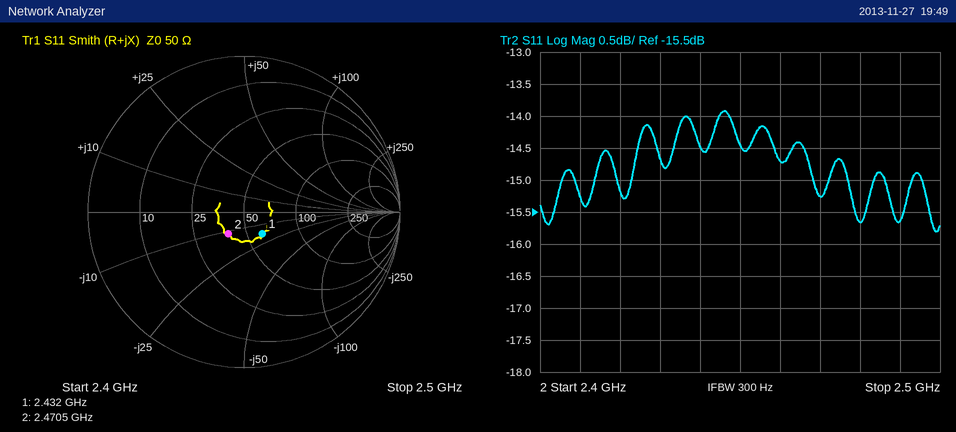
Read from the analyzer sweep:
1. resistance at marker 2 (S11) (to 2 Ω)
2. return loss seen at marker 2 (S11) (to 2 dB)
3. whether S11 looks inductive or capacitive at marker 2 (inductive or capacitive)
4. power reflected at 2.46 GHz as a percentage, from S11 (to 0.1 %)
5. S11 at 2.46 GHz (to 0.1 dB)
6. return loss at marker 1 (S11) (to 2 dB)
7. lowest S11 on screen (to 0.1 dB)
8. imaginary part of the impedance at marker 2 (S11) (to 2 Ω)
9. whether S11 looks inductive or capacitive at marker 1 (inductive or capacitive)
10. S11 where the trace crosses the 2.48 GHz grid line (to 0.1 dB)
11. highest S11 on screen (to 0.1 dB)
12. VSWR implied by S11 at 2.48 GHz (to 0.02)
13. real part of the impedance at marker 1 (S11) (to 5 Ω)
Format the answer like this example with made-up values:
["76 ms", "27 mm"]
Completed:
["40 Ω", "16 dB", "capacitive", "3.4 %", "-14.7 dB", "14 dB", "-15.8 dB", "-12 Ω", "capacitive", "-15.7 dB", "-13.9 dB", "1.40", "60 Ω"]
